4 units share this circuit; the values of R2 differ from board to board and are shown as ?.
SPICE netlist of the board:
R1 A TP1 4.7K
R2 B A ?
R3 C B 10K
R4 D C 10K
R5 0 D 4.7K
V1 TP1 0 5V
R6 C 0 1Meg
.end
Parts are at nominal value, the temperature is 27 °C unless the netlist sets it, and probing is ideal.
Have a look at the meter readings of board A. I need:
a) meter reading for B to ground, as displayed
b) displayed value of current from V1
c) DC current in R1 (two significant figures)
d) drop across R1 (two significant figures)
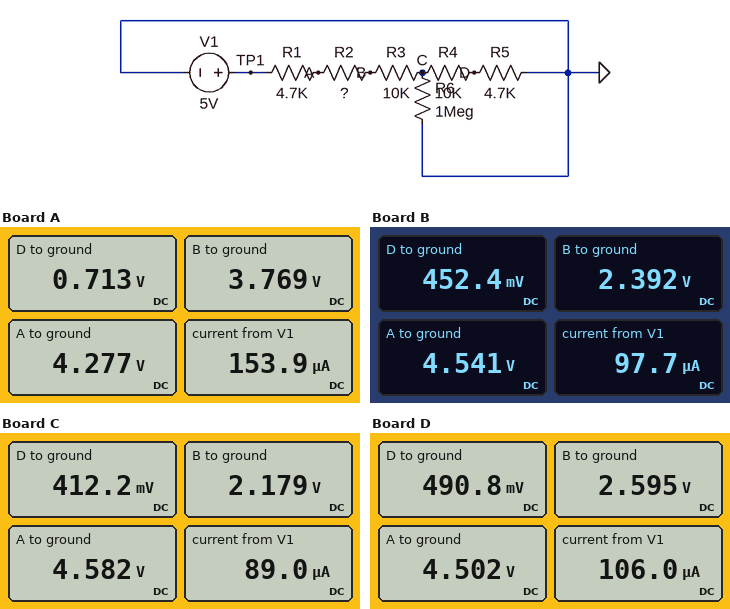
3.769 V
153.9 µA
150 µA
720 mV
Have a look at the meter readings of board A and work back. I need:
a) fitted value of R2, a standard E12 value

3.3 kΩ
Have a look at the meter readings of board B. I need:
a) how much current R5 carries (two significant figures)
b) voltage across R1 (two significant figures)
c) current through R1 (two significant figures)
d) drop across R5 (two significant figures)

96 µA
460 mV
98 µA
450 mV
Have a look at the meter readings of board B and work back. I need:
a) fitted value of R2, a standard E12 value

22 kΩ
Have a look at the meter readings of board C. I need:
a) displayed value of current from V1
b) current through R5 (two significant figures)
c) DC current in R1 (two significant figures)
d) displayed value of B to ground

89.0 µA
88 µA
89 µA
2.179 V
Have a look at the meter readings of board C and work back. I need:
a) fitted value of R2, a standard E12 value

27 kΩ
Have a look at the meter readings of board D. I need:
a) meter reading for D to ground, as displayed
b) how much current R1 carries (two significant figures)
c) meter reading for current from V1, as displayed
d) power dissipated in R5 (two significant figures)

490.8 mV
110 µA
106.0 µA
51 µW
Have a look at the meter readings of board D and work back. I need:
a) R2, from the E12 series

18 kΩ
